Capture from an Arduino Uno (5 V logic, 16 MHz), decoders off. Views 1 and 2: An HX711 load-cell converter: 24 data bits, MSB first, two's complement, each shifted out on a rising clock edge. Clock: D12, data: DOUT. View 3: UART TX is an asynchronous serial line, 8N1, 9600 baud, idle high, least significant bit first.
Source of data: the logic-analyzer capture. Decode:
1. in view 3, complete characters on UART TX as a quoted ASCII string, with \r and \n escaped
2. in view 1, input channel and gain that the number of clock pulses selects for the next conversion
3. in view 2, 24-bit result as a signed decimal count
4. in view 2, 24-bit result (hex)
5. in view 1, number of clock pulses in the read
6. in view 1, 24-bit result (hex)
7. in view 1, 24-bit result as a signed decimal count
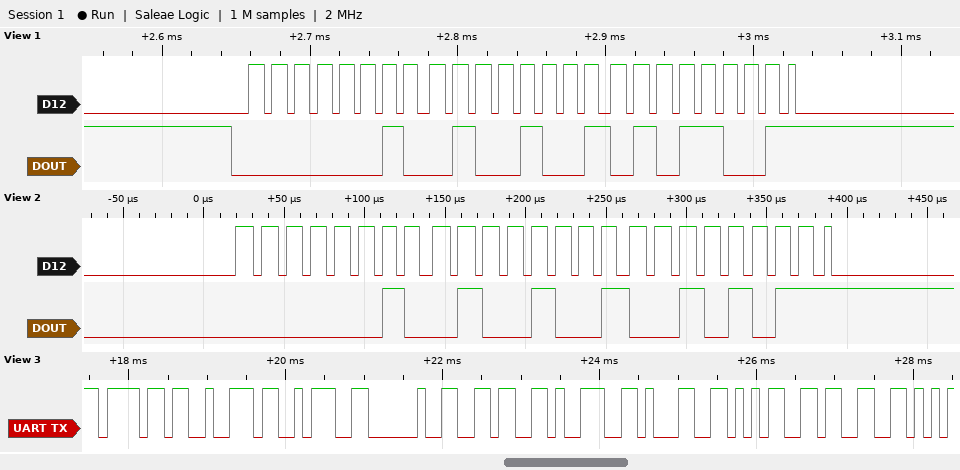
"or: 69153"
channel A, gain 128
149803
0x02492B
25
0x024959
149849
